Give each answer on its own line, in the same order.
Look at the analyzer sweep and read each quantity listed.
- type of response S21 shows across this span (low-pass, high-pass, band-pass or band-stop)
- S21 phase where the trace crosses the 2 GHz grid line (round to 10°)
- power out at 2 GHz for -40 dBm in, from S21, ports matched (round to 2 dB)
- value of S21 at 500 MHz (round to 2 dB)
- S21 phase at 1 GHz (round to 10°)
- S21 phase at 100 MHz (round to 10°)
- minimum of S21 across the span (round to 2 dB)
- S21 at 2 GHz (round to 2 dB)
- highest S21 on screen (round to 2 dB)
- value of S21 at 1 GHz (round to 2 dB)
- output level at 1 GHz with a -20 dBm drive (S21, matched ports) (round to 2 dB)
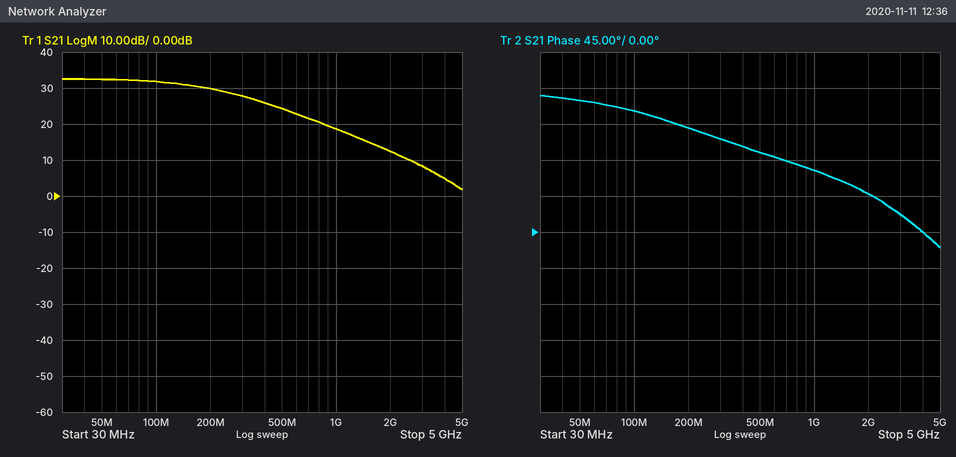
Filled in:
low-pass
50°
-28 dBm
24 dB
80°
150°
2 dB
12 dB
32 dB
18 dB
-2 dBm
